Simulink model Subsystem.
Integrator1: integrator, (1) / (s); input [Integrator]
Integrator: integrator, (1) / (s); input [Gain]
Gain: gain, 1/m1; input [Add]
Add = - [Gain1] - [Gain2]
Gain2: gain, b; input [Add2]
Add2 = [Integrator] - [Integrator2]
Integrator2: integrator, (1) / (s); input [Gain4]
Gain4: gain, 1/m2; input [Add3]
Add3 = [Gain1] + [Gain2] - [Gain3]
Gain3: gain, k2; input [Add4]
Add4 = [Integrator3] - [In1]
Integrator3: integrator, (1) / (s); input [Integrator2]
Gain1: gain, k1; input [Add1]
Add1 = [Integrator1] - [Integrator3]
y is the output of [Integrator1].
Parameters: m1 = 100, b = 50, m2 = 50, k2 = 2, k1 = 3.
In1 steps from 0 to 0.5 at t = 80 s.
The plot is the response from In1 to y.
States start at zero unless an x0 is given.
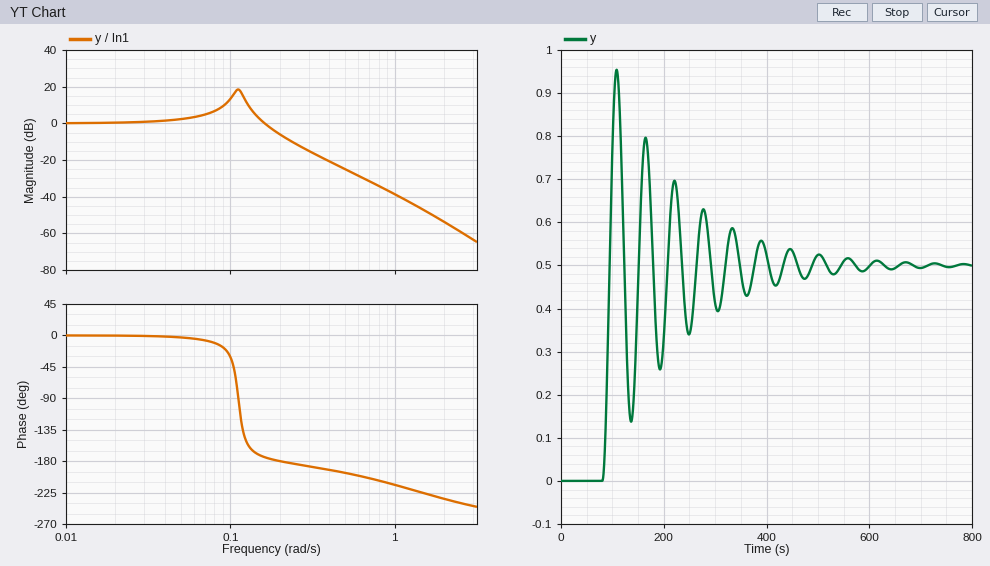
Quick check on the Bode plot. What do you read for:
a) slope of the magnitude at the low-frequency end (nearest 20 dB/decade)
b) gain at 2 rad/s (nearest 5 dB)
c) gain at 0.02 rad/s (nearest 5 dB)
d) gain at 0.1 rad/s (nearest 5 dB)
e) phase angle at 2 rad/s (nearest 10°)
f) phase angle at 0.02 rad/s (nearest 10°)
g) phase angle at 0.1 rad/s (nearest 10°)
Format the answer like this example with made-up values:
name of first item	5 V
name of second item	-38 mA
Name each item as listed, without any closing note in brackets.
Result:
slope of the magnitude at the low-frequency end	0 dB/decade
gain at 2 rad/s	-55 dB
gain at 0.02 rad/s	0 dB
gain at 0.1 rad/s	15 dB
phase angle at 2 rad/s	-230°
phase angle at 0.02 rad/s	0°
phase angle at 0.1 rad/s	-30°
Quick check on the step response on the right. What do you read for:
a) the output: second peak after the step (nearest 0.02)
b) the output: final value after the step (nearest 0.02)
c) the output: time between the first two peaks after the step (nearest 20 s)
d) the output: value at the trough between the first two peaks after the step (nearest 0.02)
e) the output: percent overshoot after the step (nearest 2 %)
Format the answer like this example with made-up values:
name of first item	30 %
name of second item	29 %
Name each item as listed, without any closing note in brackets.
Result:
the output: second peak after the step	0.80
the output: final value after the step	0.50
the output: time between the first two peaks after the step	60 s
the output: value at the trough between the first two peaks after the step	0.14
the output: percent overshoot after the step	90 %
